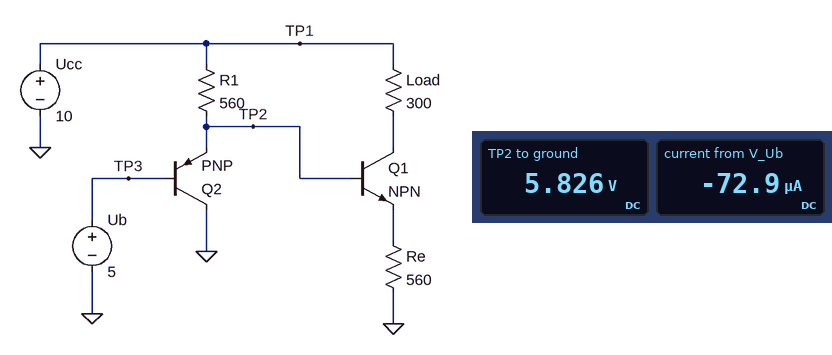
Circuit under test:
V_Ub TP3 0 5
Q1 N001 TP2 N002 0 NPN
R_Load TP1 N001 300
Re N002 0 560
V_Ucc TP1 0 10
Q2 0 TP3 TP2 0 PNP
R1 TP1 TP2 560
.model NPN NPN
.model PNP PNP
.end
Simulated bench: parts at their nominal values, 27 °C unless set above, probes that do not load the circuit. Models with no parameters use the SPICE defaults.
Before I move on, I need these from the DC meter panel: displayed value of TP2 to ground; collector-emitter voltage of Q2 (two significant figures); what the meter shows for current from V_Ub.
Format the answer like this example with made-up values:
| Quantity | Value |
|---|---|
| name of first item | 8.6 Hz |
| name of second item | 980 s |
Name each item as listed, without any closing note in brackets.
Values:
| Quantity | Value |
|---|---|
| displayed value of TP2 to ground | 5.826 V |
| collector-emitter voltage of Q2 | -5.8 V |
| what the meter shows for current from V_Ub | -72.9 µA |
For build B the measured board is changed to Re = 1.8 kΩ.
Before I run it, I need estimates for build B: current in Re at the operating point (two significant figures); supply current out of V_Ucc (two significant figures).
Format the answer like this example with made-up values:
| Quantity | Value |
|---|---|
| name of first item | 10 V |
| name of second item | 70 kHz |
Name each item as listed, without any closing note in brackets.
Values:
| Quantity | Value |
|---|---|
| current in Re at the operating point | 2.8 mA |
| supply current out of V_Ucc | 10 mA |
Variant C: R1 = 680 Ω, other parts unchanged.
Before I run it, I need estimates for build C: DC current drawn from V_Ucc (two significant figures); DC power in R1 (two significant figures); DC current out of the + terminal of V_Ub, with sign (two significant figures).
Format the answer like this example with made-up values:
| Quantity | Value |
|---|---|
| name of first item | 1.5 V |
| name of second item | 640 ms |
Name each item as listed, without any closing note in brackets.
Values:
| Quantity | Value |
|---|---|
| DC current drawn from V_Ucc | 15 mA |
| DC power in R1 | 26 mW |
| DC current out of the + terminal of V_Ub, with sign | -60 µA |
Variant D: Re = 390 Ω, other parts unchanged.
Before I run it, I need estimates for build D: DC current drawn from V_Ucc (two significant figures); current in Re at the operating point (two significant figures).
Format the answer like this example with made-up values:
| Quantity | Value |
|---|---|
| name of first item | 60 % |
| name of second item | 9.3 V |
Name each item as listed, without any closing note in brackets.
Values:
| Quantity | Value |
|---|---|
| DC current drawn from V_Ucc | 20 mA |
| current in Re at the operating point | 13 mA |
